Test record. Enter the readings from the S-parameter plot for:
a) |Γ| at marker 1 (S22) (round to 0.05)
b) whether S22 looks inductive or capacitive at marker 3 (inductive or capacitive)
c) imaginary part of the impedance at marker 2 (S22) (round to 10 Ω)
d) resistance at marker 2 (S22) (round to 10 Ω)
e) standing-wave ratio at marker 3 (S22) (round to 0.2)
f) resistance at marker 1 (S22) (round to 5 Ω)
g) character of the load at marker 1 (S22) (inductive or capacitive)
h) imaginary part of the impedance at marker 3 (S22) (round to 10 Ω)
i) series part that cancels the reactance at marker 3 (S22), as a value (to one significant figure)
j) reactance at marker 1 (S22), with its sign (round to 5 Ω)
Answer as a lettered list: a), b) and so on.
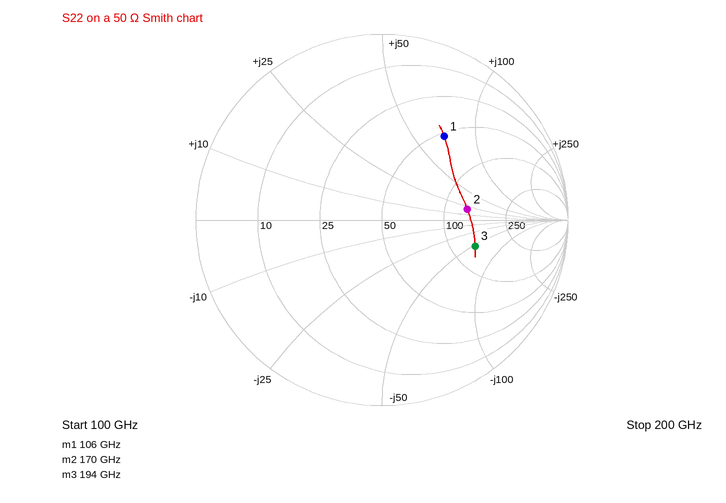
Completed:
a) 0.55
b) capacitive
c) +20 Ω
d) 130 Ω
e) 3.2
f) 55 Ω
g) inductive
h) -50 Ω
i) 40 pH
j) +70 Ω
